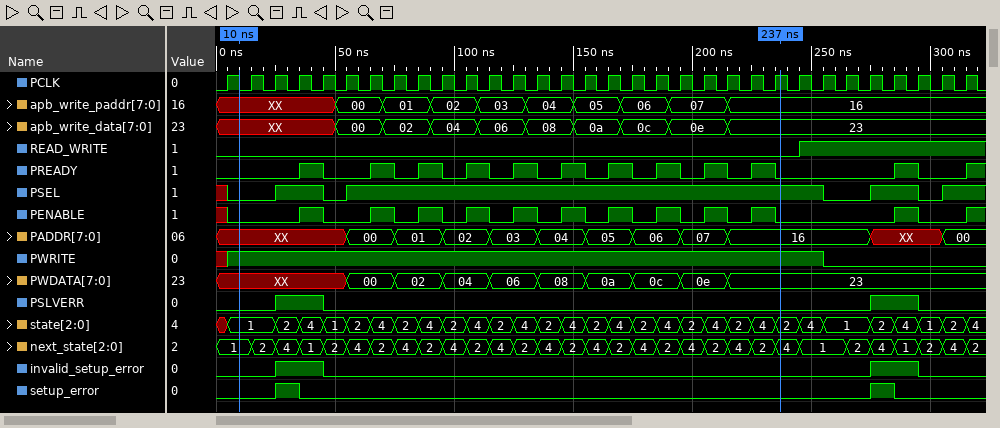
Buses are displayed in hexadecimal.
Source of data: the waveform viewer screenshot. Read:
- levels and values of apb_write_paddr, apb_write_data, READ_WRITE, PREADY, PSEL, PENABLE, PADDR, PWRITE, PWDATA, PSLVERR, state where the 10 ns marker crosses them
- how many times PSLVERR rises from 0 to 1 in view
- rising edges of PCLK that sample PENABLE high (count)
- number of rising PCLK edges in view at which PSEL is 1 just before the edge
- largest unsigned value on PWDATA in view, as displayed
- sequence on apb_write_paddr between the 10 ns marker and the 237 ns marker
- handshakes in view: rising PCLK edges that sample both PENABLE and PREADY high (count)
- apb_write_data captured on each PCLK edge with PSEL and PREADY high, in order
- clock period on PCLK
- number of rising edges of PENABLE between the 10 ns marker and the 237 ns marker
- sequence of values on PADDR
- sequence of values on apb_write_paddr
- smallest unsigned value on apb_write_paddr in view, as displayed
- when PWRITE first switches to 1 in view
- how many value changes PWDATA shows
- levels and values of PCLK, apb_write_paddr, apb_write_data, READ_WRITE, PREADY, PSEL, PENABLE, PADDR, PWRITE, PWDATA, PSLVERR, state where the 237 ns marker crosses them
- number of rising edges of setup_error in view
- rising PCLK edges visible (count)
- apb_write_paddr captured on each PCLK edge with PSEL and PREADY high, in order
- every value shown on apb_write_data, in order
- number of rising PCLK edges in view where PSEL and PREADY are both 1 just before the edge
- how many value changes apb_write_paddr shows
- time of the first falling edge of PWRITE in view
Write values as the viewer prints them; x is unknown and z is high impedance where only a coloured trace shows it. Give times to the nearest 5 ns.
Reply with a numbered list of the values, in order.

1. apb_write_paddr=XX, apb_write_data=XX, READ_WRITE=0, PREADY=0, PSEL=0, PENABLE=0, PADDR=XX, PWRITE=1, PWDATA=XX, PSLVERR=0, state=1
2. 2
3. 11
4. 25
5. 23
6. XX, 00, 01, 02, 03, 04, 05, 06, 07, 16
7. 11
8. XX, 02, 04, 06, 08, 0a, 0c, 0e, 0e, 23, 23
9. 10 ns
10. 10
11. XX, 00, 01, 02, 03, 04, 05, 06, 07, 16, XX, 00
12. XX, 00, 01, 02, 03, 04, 05, 06, 07, 16
13. 00
14. 5 ns
15. 9
16. PCLK=1, apb_write_paddr=16, apb_write_data=23, READ_WRITE=0, PREADY=0, PSEL=1, PENABLE=0, PADDR=16, PWRITE=1, PWDATA=23, PSLVERR=0, state=2
17. 2
18. 32
19. XX, 01, 02, 03, 04, 05, 06, 07, 07, 16, 16
20. XX, 00, 02, 04, 06, 08, 0a, 0c, 0e, 23
21. 11
22. 9
23. 255 ns
